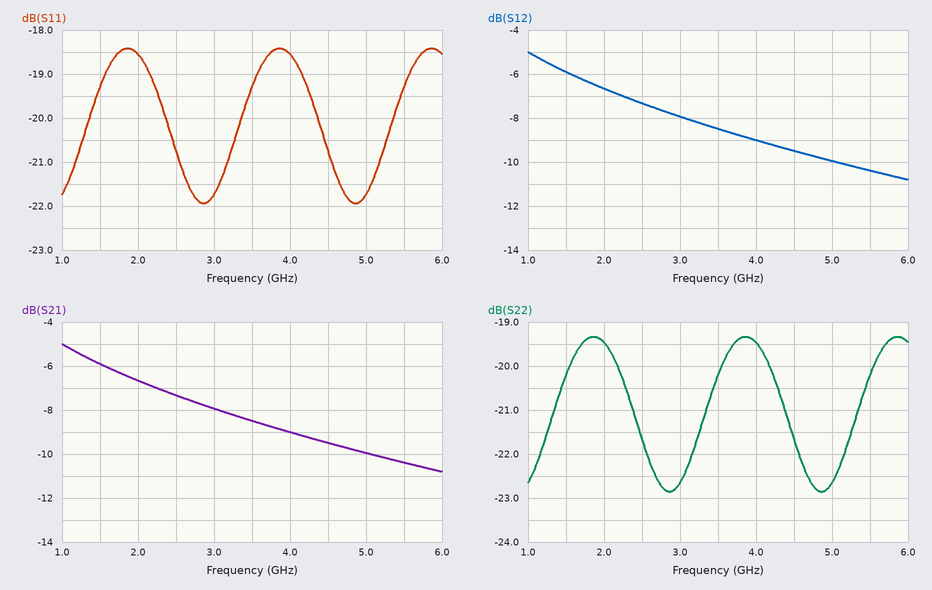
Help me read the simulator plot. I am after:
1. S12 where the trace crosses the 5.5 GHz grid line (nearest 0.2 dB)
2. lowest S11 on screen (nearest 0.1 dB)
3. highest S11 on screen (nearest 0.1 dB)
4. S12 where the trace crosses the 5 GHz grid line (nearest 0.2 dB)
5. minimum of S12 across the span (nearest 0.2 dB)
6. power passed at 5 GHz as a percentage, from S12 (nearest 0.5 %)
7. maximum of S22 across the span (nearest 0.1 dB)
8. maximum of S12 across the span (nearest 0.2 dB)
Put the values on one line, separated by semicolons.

-10.4 dB; -21.9 dB; -18.4 dB; -10.0 dB; -10.8 dB; 10.0 %; -19.3 dB; -5.0 dB
